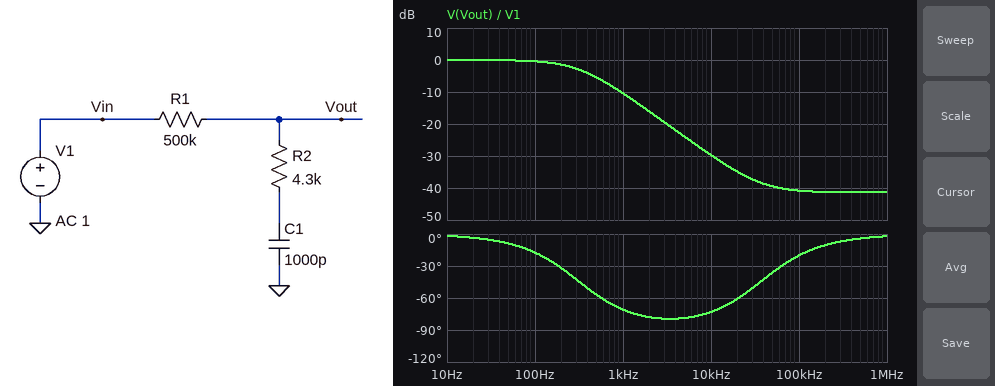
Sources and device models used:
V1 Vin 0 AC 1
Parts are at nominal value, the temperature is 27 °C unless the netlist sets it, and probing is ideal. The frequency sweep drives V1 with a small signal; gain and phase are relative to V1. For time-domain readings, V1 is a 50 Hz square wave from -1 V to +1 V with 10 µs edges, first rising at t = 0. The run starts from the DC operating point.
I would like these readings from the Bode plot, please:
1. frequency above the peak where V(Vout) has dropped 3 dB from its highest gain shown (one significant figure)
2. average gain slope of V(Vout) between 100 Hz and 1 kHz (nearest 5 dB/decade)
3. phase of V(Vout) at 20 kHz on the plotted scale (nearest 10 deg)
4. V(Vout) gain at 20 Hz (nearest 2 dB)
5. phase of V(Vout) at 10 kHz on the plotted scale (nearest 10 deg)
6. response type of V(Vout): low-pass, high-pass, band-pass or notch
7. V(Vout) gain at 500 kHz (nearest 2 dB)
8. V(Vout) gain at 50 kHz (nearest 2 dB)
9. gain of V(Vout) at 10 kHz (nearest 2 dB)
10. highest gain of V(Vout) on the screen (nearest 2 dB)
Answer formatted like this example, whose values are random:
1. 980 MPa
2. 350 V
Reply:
1. 300 Hz
2. -10 dB/decade
3. -60 deg
4. 0 dB
5. -70 deg
6. low-pass
7. -42 dB
8. -40 dB
9. -30 dB
10. 0 dB
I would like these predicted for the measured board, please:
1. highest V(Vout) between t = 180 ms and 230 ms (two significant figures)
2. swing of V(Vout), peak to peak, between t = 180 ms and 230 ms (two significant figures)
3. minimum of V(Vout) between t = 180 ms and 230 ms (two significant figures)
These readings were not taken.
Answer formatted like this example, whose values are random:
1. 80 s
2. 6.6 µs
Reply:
1. 1.0 V
2. 2.0 V
3. -1.0 V
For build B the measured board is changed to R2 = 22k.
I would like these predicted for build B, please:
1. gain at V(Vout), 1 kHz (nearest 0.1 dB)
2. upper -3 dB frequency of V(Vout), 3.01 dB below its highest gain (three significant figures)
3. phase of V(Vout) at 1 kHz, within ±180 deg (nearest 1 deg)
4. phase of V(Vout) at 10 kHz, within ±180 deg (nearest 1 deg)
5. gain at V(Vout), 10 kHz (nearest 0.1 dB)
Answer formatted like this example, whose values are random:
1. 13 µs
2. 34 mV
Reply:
1. -10.6 dB
2. 305 Hz
3. -65 deg
4. -34 deg
5. -25.7 dB
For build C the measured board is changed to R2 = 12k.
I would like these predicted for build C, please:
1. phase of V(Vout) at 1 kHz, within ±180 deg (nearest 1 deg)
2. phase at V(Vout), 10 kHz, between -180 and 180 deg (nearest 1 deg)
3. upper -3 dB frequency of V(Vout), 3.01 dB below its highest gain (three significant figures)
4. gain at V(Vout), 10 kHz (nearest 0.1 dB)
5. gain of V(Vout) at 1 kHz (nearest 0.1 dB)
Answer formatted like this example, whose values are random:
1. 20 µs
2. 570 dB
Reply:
1. -68 deg
2. -51 deg
3. 311 Hz
4. -28.2 dB
5. -10.5 dB
